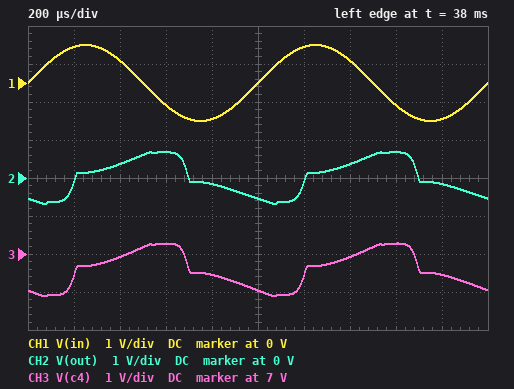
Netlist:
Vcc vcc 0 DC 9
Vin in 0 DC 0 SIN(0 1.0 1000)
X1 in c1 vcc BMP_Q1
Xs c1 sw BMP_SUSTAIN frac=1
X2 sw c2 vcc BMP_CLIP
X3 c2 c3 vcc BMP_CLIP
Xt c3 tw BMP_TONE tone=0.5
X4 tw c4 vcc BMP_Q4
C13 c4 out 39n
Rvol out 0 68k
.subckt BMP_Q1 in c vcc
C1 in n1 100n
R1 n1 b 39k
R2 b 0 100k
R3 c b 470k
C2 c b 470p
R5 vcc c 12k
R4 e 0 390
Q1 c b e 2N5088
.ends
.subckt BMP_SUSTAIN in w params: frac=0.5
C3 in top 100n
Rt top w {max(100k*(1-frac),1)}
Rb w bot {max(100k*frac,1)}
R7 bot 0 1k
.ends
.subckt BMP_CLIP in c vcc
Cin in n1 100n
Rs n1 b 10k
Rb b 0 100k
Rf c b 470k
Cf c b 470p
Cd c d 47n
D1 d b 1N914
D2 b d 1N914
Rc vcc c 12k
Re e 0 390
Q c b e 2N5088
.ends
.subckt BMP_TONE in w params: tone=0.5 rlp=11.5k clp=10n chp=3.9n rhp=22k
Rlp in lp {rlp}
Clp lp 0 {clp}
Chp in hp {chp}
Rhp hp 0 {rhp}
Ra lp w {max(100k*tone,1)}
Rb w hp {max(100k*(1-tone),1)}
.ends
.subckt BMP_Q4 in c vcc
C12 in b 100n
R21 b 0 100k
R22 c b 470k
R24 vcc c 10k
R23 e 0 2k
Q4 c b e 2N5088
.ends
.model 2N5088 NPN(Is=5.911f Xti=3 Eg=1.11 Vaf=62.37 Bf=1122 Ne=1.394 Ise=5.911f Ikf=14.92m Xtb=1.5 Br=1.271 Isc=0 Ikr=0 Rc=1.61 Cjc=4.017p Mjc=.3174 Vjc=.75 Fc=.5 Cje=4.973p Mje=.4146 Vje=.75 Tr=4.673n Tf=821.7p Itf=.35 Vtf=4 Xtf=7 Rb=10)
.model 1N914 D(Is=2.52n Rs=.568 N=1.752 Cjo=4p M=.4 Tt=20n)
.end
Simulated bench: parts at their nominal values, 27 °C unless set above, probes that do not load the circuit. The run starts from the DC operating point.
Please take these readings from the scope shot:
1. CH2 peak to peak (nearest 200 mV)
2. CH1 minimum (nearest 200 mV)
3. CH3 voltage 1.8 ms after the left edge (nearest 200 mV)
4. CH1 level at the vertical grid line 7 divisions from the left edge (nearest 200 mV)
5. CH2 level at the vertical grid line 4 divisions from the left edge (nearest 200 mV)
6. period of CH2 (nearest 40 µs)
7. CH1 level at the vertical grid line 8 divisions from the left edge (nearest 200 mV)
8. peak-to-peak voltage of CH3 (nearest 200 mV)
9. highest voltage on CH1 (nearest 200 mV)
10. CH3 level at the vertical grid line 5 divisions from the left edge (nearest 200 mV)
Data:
1.4 V
-1.0 V
6.4 V
600 mV
-200 mV
1.00 ms
-600 mV
1.4 V
1.0 V
6.0 V
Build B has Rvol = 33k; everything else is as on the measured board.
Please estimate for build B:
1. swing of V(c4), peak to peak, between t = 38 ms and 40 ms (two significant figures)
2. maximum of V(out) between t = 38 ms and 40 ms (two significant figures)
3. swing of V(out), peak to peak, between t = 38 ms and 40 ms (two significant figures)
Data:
1.3 V
600 mV
1.2 V
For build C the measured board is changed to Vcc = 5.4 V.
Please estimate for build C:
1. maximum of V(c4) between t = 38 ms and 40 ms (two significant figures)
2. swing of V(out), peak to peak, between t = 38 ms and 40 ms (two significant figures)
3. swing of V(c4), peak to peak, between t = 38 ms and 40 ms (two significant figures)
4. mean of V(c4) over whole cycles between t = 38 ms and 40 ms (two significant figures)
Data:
5.0 V
940 mV
970 mV
4.6 V
